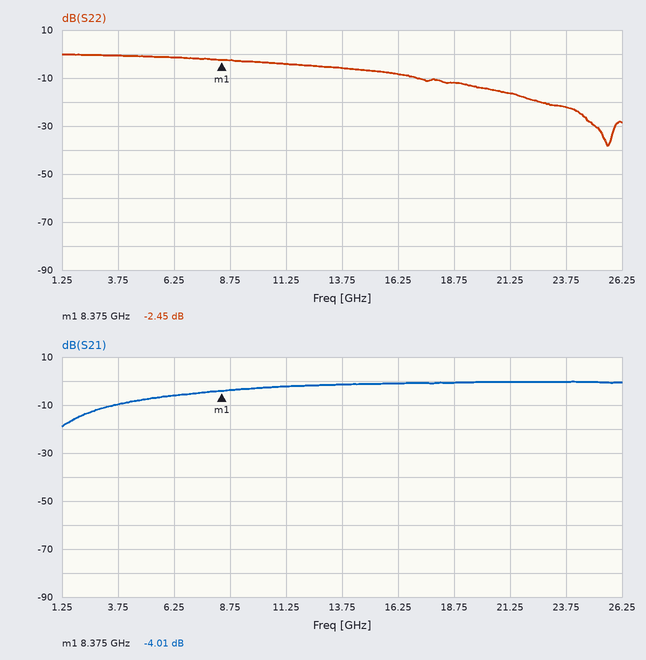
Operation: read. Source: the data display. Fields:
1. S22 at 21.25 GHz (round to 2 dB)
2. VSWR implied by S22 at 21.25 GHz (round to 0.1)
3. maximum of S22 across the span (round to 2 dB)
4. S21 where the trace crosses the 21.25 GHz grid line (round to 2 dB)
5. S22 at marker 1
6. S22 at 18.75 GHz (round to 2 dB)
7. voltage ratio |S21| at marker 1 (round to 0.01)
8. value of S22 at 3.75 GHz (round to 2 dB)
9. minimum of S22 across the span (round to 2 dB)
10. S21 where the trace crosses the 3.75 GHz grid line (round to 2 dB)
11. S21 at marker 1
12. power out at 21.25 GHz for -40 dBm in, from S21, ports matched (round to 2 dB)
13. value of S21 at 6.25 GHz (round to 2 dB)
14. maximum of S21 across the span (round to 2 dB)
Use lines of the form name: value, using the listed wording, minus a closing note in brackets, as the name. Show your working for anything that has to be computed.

S22 at 21.25 GHz: -16 dB
VSWR implied by S22 at 21.25 GHz: |Γ| = 10^(-16/20) = 0.1585; VSWR = (1 + 0.1585)/(1 − 0.1585) ≈ 1.4
maximum of S22 across the span: 0 dB
S21 where the trace crosses the 21.25 GHz grid line: 0 dB
S22 at marker 1: -2.45 dB
S22 at 18.75 GHz: -12 dB
voltage ratio |S21| at marker 1: 10^(-4.01/20) ≈ 0.63
value of S22 at 3.75 GHz: 0 dB
minimum of S22 across the span: -38 dB
S21 where the trace crosses the 3.75 GHz grid line: -10 dB
S21 at marker 1: -4.01 dB
power out at 21.25 GHz for -40 dBm in, from S21, ports matched: -40 dBm + (0 dB) = -40 dBm
value of S21 at 6.25 GHz: -6 dB
maximum of S21 across the span: 0 dB
